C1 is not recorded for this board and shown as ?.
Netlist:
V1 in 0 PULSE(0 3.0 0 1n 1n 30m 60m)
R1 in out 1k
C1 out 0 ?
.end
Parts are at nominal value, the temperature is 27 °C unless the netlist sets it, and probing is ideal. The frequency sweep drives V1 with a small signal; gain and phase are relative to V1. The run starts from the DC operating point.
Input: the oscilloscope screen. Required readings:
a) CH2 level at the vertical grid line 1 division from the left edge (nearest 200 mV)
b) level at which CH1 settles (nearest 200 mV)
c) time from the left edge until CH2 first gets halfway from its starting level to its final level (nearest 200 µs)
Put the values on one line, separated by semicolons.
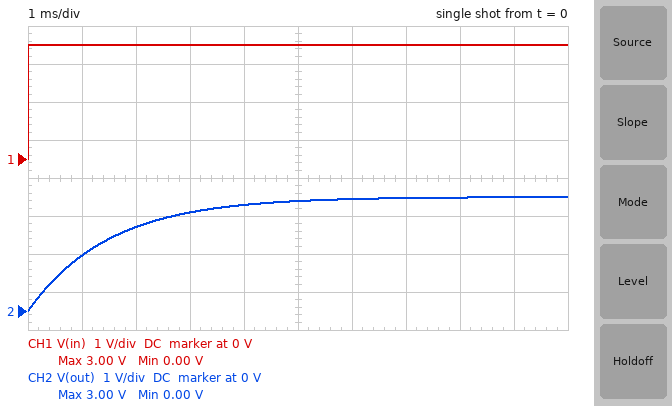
1.4 V; 3.0 V; 1.0 ms
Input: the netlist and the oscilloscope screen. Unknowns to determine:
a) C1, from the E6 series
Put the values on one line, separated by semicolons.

1.5 µF
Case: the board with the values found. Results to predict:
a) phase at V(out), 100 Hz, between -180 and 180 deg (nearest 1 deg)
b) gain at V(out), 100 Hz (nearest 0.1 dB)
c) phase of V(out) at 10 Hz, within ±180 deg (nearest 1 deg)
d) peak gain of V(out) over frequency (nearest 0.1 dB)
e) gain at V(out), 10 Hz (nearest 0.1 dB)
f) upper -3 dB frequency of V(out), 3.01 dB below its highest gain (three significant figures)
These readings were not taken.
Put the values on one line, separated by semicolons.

-43 deg; -2.8 dB; -5 deg; 0 dB; 0 dB; 106 Hz
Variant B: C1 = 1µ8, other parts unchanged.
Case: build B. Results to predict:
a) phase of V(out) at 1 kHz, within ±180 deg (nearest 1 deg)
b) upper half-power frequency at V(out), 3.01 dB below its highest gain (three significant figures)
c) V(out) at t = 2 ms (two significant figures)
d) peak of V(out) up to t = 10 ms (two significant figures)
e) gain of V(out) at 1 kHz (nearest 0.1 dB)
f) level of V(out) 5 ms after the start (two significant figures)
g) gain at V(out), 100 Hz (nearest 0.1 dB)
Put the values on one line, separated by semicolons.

-85 deg; 88.4 Hz; 2.0 V; 3.0 V; -21.1 dB; 2.8 V; -3.6 dB
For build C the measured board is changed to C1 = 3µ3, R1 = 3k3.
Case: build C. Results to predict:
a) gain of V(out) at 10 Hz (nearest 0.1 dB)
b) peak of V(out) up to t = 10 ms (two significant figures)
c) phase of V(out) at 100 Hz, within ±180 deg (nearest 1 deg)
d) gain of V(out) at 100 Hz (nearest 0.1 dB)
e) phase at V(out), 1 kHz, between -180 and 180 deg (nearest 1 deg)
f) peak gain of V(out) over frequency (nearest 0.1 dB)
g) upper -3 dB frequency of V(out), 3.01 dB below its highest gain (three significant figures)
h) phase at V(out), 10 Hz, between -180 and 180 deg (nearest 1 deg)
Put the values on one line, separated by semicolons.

-1.7 dB; 1.8 V; -82 deg; -16.8 dB; -89 deg; 0 dB; 14.6 Hz; -34 deg
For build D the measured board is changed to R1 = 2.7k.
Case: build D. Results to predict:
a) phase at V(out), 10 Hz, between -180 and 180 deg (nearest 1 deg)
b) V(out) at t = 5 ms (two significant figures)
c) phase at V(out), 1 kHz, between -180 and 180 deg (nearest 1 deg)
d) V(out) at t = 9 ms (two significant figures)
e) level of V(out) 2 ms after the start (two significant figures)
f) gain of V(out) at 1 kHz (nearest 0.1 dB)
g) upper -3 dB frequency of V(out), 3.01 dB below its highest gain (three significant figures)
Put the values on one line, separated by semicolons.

-14 deg; 2.1 V; -88 deg; 2.7 V; 1.2 V; -28.1 dB; 39.3 Hz
